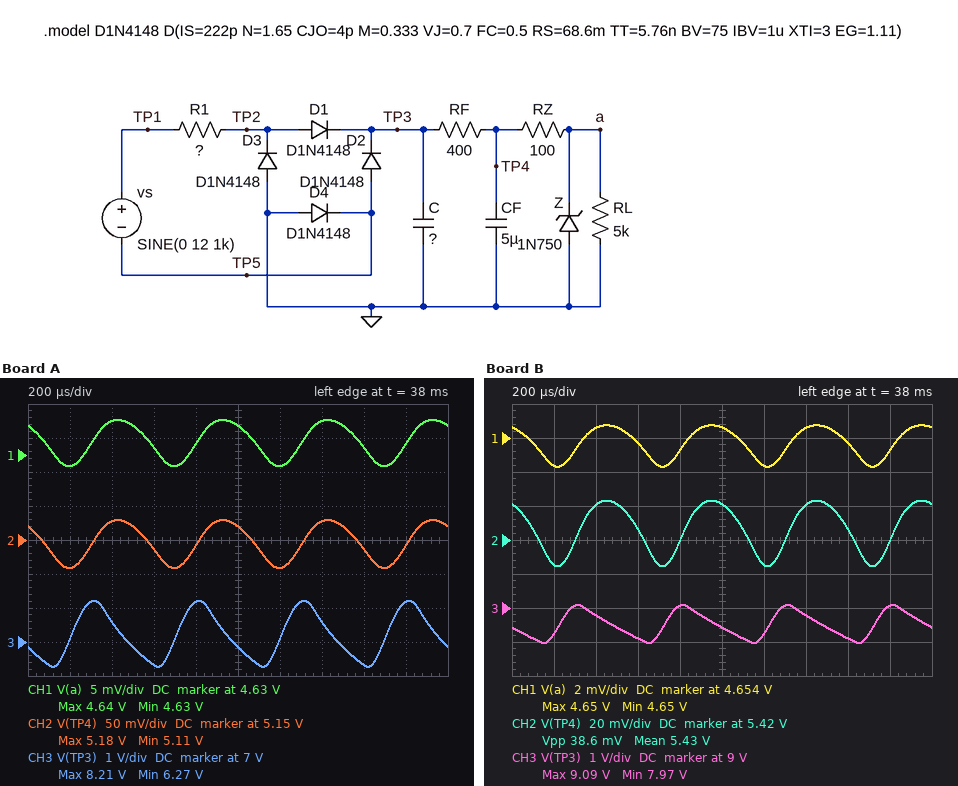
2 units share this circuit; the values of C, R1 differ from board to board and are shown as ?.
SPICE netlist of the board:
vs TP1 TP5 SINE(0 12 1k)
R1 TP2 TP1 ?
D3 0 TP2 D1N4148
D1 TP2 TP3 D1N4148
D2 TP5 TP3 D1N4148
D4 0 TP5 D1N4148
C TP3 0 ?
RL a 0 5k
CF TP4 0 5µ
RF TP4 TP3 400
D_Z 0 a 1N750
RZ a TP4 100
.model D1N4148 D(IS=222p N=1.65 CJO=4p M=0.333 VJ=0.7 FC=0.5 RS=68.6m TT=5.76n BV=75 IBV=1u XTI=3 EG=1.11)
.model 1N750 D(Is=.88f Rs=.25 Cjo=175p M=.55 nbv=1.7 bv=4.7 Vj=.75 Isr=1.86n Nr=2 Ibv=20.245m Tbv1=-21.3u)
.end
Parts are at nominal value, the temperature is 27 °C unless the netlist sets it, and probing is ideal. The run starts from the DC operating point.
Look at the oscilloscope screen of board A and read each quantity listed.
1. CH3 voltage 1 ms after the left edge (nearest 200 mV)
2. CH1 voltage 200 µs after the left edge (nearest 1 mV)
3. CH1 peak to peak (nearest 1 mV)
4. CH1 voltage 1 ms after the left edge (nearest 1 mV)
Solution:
6.8 V
4.628 V
7 mV
4.634 V
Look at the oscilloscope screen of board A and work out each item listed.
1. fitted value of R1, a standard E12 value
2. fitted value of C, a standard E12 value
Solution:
180 Ω
680 nF
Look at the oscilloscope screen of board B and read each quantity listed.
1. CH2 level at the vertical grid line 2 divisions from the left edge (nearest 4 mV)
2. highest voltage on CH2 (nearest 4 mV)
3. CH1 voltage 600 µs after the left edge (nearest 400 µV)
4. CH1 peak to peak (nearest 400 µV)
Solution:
5.440 V
5.444 V
4.6536 V
2.4 mV
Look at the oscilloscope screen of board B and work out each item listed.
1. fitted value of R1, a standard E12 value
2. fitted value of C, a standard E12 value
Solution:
56 Ω
2.2 µF
